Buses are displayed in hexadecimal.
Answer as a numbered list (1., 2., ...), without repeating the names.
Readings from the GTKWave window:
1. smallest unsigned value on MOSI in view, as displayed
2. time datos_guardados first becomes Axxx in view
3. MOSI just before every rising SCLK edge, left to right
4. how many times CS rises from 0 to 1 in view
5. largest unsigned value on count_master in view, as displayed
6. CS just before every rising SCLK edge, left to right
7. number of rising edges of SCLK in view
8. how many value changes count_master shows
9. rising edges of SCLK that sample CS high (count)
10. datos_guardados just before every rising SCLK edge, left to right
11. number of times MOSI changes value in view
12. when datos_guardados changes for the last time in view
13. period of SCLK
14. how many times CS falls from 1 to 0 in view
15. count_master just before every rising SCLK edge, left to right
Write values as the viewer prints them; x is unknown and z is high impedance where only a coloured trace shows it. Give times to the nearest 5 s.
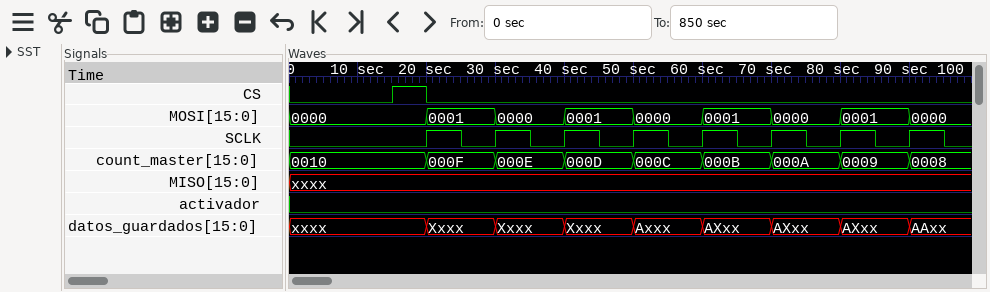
1. 0000
2. 50 s
3. 0000, 0001, 0000, 0001, 0000, 0001, 0000, 0001
4. 1
5. 0010
6. 1 0 0 0 0 0 0 0
7. 8
8. 8
9. 1
10. xxxx, Xxxx, Xxxx, Xxxx, Axxx, AXxx, AXxx, AXxx
11. 8
12. 90 s
13. 10 s
14. 1
15. 0010, 000F, 000E, 000D, 000C, 000B, 000A, 0009
